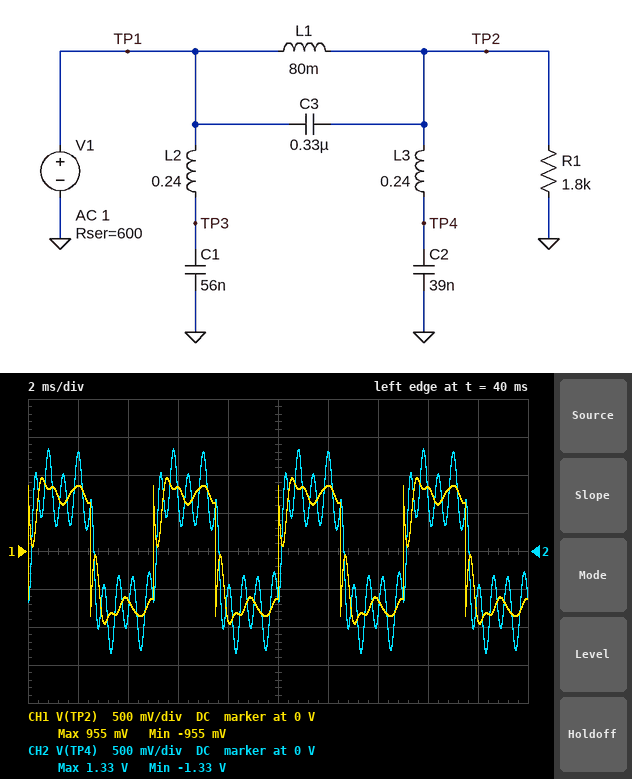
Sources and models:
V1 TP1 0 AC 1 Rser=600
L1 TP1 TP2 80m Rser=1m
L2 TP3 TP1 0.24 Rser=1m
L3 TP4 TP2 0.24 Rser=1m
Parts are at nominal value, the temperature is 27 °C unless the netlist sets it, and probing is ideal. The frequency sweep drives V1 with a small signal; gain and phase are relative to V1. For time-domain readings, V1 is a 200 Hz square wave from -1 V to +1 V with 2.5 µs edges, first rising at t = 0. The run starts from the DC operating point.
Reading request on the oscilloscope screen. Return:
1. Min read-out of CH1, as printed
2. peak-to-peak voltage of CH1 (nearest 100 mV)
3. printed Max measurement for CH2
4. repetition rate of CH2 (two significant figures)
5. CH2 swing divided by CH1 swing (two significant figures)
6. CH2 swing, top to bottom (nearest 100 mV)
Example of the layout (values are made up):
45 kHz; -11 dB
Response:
-955 mV; 1.9 V; 1.33 V; 200 Hz; 1.4; 2.7 V
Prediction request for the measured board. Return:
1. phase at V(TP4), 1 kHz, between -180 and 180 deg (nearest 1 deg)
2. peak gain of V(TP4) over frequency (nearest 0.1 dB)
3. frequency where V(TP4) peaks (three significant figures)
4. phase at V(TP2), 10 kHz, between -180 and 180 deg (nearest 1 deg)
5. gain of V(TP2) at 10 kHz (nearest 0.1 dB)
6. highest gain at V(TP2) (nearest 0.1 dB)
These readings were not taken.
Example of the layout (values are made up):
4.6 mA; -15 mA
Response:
23 deg; 13.8 dB; 1.66 kHz; 5 deg; -2.5 dB; -2.3 dB
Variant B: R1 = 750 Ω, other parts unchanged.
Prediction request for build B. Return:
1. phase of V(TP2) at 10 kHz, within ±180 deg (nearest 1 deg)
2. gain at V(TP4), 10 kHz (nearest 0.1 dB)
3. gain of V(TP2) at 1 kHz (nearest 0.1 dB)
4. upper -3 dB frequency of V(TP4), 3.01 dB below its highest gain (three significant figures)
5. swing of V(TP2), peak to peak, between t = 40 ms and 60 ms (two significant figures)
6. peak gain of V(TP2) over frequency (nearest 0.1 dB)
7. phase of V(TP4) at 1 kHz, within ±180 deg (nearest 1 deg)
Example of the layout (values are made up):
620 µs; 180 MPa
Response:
5 deg; -36.2 dB; -25.5 dB; 1.74 kHz; 1.4 V; -5.1 dB; 44 deg
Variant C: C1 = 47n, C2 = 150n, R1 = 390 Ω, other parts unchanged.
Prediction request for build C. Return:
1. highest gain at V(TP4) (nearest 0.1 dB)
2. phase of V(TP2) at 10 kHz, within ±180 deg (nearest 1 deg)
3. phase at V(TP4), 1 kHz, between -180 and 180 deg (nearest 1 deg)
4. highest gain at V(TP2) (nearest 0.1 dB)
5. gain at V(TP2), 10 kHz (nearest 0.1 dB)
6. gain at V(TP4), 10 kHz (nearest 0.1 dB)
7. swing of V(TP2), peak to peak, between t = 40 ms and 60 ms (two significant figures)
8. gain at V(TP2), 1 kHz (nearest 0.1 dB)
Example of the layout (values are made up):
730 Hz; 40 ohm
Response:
1.5 dB; 5 deg; -70 deg; -7.9 dB; -8.1 dB; -51.1 dB; 1.0 V; -32.6 dB
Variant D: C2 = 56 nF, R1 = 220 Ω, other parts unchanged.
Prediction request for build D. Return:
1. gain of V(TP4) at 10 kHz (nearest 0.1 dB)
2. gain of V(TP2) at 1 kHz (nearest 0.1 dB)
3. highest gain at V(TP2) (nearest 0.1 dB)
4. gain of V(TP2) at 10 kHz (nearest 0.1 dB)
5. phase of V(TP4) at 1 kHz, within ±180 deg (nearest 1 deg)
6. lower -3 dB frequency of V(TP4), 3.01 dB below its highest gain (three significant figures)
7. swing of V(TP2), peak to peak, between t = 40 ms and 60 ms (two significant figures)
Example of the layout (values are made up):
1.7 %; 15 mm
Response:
-45.8 dB; -35.8 dB; -10.8 dB; -11.4 dB; 53 deg; 1.43 kHz; 660 mV
